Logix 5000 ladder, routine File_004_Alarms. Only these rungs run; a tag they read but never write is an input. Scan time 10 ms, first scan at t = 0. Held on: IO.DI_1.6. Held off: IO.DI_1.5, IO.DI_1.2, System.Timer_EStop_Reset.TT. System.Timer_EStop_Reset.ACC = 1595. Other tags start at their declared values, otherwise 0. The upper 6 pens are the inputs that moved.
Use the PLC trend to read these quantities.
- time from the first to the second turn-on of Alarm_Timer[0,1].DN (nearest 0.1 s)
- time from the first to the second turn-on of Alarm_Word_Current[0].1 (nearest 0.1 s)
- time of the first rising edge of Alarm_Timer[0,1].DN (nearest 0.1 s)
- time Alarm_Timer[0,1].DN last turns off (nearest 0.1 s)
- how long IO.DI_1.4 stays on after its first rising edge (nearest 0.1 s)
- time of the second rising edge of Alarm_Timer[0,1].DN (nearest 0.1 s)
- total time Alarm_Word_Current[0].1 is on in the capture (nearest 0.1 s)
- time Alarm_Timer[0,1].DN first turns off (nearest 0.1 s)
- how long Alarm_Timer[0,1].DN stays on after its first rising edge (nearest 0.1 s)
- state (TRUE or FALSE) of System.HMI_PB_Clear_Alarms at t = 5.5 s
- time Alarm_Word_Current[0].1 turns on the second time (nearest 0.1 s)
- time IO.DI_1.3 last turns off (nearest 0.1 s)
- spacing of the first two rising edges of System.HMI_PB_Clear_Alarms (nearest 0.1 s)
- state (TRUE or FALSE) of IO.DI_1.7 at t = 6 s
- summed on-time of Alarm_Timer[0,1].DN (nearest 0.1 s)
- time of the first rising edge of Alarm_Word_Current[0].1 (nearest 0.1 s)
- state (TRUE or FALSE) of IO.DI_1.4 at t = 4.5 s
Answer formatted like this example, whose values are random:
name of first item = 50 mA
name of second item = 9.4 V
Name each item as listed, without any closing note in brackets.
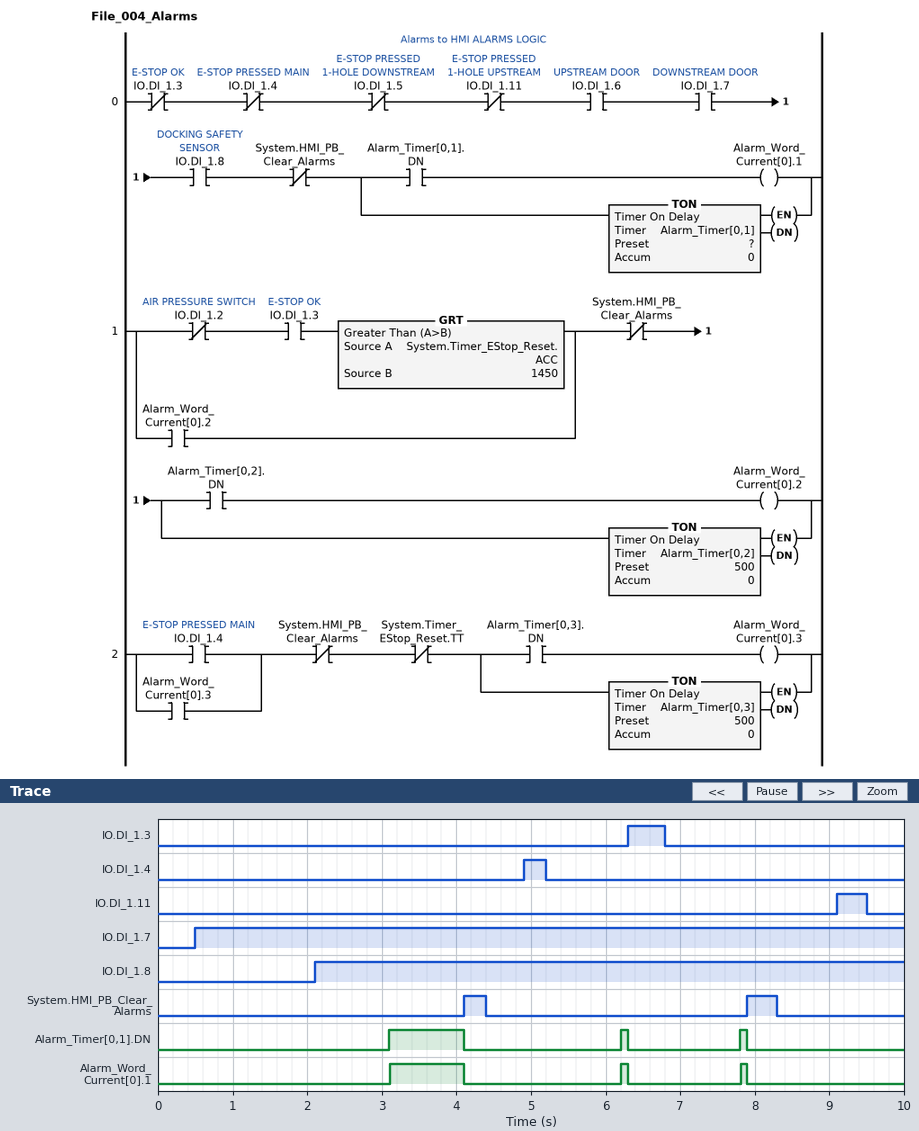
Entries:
time from the first to the second turn-on of Alarm_Timer[0,1].DN = 3.1 s
time from the first to the second turn-on of Alarm_Word_Current[0].1 = 3.1 s
time of the first rising edge of Alarm_Timer[0,1].DN = 3.1 s
time Alarm_Timer[0,1].DN last turns off = 7.9 s
how long IO.DI_1.4 stays on after its first rising edge = 0.3 s
time of the second rising edge of Alarm_Timer[0,1].DN = 6.2 s
total time Alarm_Word_Current[0].1 is on in the capture = 1.2 s
time Alarm_Timer[0,1].DN first turns off = 4.1 s
how long Alarm_Timer[0,1].DN stays on after its first rising edge = 1.0 s
state (TRUE or FALSE) of System.HMI_PB_Clear_Alarms at t = 5.5 s = FALSE
time Alarm_Word_Current[0].1 turns on the second time = 6.2 s
time IO.DI_1.3 last turns off = 6.8 s
spacing of the first two rising edges of System.HMI_PB_Clear_Alarms = 3.8 s
state (TRUE or FALSE) of IO.DI_1.7 at t = 6 s = TRUE
summed on-time of Alarm_Timer[0,1].DN = 1.2 s
time of the first rising edge of Alarm_Word_Current[0].1 = 3.1 s
state (TRUE or FALSE) of IO.DI_1.4 at t = 4.5 s = FALSE
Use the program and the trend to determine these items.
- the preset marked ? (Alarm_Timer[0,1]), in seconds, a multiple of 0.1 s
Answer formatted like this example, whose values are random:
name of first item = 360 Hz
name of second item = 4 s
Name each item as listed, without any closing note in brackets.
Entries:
the preset marked ? (Alarm_Timer[0,1]), in seconds, a multiple of 0.1 s = 1.0 s
